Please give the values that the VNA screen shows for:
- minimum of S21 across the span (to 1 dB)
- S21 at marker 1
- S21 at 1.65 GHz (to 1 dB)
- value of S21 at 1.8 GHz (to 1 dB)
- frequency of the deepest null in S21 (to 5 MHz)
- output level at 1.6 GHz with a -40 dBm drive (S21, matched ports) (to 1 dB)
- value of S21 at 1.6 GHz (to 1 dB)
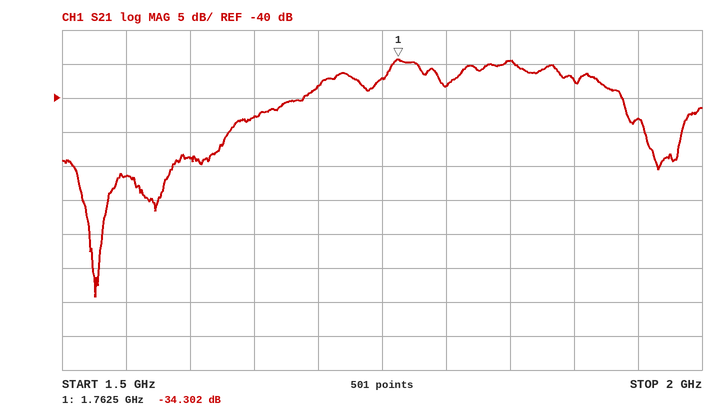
-69 dB
-34.302 dB
-43 dB
-38 dB
1.525 GHz
-89 dBm
-49 dB
